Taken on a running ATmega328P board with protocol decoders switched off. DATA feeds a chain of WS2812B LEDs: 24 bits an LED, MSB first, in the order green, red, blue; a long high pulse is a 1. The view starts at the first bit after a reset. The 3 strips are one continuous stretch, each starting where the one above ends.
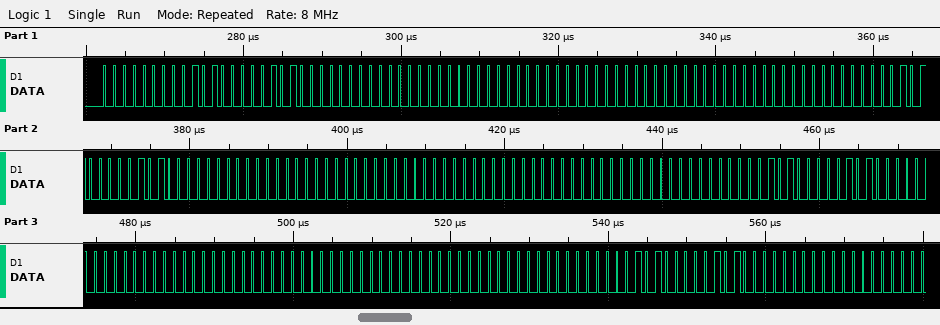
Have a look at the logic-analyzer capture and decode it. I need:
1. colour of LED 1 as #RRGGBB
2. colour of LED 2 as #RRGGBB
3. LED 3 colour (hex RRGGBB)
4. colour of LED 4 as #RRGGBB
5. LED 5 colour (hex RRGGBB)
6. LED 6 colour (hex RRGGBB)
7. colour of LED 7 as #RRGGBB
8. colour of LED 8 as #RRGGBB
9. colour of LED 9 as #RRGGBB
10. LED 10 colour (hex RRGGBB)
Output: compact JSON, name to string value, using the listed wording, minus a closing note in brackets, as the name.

{"colour of LED 1 as #RRGGBB": "#500050", "colour of LED 2 as #RRGGBB": "#000000", "LED 3 colour": "#000000", "colour of LED 4 as #RRGGBB": "#500050", "LED 5 colour": "#000000", "LED 6 colour": "#000000", "colour of LED 7 as #RRGGBB": "#500050", "colour of LED 8 as #RRGGBB": "#000000", "colour of LED 9 as #RRGGBB": "#000000", "LED 10 colour": "#500050"}
